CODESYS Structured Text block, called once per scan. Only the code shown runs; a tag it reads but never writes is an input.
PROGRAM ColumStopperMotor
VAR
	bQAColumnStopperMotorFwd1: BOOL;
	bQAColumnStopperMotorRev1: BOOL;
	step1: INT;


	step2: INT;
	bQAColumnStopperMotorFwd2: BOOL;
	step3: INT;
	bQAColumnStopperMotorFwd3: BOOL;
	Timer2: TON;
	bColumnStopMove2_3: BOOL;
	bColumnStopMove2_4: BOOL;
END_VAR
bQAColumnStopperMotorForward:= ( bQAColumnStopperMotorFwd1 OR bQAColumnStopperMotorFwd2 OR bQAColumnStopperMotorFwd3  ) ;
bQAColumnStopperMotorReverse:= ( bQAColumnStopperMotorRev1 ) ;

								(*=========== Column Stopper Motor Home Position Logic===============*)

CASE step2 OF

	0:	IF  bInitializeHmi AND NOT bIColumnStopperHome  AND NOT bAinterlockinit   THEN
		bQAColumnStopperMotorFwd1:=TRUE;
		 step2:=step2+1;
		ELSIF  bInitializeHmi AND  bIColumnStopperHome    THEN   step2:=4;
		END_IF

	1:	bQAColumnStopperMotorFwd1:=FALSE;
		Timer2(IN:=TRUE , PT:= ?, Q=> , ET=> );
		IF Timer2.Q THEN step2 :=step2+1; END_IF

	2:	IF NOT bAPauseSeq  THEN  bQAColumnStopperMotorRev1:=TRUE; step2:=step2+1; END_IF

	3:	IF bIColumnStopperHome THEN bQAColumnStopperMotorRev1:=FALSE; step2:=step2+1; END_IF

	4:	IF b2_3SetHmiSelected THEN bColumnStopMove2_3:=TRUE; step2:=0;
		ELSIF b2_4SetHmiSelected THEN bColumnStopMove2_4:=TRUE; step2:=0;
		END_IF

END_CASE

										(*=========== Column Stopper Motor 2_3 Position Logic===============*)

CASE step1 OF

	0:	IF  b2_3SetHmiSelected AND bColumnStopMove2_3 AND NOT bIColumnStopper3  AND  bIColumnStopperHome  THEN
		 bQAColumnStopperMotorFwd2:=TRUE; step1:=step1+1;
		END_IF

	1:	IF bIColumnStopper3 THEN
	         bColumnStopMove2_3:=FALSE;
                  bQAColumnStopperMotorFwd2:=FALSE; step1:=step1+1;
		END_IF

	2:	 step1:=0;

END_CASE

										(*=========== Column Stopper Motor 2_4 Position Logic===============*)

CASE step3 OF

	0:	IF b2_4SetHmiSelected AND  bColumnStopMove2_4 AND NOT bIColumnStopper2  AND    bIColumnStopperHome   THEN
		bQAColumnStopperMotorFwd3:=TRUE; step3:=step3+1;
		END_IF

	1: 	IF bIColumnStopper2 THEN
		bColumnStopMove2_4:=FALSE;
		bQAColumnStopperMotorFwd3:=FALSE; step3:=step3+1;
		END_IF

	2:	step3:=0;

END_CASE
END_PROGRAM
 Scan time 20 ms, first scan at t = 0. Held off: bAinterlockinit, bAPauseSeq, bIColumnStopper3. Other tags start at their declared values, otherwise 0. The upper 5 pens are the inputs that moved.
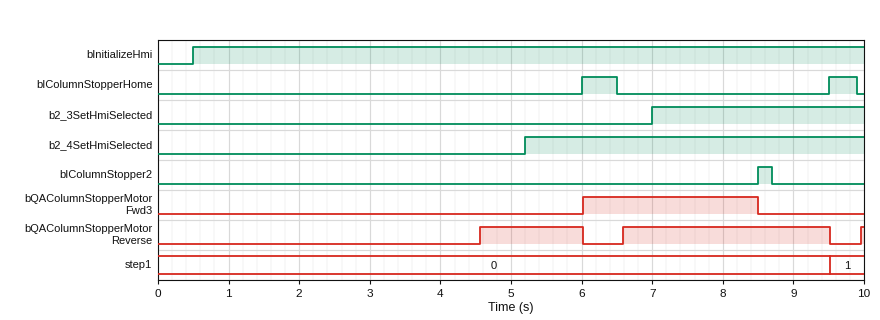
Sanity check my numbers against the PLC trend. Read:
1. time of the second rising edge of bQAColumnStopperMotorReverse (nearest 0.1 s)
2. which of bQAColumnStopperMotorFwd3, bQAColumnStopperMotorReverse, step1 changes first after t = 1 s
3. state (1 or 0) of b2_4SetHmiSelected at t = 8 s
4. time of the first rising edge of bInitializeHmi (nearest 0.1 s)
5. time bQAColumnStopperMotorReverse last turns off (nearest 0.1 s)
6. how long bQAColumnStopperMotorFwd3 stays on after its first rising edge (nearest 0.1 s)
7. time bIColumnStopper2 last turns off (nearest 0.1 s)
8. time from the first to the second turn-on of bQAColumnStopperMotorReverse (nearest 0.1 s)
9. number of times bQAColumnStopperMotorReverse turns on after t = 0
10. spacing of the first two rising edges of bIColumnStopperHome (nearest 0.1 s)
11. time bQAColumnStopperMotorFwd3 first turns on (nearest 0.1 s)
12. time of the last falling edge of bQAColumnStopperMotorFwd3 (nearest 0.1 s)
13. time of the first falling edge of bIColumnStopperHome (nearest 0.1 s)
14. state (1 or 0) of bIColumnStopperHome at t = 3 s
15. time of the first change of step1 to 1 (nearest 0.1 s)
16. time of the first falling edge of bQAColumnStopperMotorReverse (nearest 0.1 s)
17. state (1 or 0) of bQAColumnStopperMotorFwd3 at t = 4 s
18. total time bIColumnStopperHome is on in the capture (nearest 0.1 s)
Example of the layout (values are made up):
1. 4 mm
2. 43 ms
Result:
1. 6.6 s
2. bQAColumnStopperMotorReverse
3. 1
4. 0.5 s
5. 9.5 s
6. 2.5 s
7. 8.7 s
8. 2.0 s
9. 3
10. 3.5 s
11. 6.0 s
12. 8.5 s
13. 6.5 s
14. 0
15. 9.5 s
16. 6.0 s
17. 0
18. 0.9 s
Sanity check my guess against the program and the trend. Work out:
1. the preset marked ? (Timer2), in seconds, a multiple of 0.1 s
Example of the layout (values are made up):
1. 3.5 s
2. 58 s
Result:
1. 4.0 s
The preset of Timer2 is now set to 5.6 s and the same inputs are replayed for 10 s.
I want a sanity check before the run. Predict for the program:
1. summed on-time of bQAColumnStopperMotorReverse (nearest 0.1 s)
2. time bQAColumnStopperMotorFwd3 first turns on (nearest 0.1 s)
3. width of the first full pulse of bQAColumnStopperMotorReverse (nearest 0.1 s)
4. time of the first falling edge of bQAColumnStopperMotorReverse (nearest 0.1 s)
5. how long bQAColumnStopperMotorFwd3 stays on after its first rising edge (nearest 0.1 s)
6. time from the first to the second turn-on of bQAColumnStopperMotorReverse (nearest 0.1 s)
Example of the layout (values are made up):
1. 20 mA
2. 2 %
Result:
1. 3.0 s
2. 6.2 s
3. 0.0 s
4. 6.2 s
5. 2.3 s
6. 0.4 s
